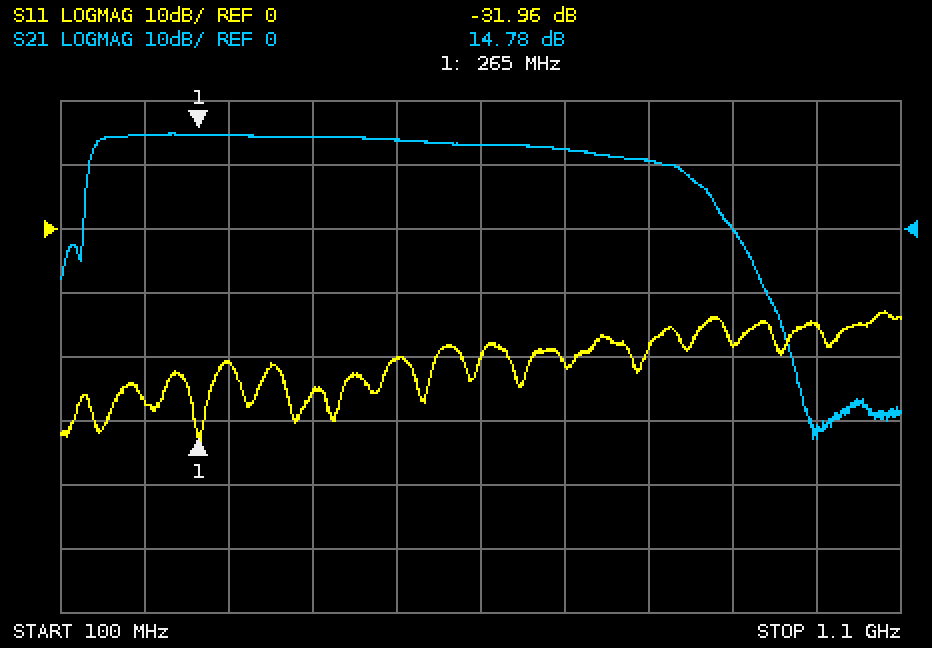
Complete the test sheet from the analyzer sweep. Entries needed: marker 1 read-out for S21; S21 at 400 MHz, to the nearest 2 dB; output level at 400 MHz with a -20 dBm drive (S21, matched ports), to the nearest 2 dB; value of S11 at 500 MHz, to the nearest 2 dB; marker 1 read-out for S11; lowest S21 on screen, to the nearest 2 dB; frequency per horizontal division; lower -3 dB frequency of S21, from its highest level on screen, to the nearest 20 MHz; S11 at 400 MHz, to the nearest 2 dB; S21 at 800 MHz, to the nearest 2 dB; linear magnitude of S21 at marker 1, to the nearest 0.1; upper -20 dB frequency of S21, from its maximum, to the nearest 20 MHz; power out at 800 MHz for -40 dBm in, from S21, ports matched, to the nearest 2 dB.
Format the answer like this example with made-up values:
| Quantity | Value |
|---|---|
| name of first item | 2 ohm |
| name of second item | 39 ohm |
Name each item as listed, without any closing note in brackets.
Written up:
| Quantity | Value |
|---|---|
| marker 1 read-out for S21 | 14.78 dB |
| S21 at 400 MHz, to the nearest 2 dB | 14 dB |
| output level at 400 MHz with a -20 dBm drive (S21, matched ports), to the nearest 2 dB | -6 dBm |
| value of S11 at 500 MHz, to the nearest 2 dB | -20 dB |
| marker 1 read-out for S11 | -31.96 dB |
| lowest S21 on screen, to the nearest 2 dB | -32 dB |
| frequency per horizontal division | 100 MHz |
| lower -3 dB frequency of S21, from its highest level on screen, to the nearest 20 MHz | 140 MHz |
| S11 at 400 MHz, to the nearest 2 dB | -26 dB |
| S21 at 800 MHz, to the nearest 2 dB | 10 dB |
| linear magnitude of S21 at marker 1, to the nearest 0.1 | 5.5 |
| upper -20 dB frequency of S21, from its maximum, to the nearest 20 MHz | 920 MHz |
| power out at 800 MHz for -40 dBm in, from S21, ports matched, to the nearest 2 dB | -30 dBm |
